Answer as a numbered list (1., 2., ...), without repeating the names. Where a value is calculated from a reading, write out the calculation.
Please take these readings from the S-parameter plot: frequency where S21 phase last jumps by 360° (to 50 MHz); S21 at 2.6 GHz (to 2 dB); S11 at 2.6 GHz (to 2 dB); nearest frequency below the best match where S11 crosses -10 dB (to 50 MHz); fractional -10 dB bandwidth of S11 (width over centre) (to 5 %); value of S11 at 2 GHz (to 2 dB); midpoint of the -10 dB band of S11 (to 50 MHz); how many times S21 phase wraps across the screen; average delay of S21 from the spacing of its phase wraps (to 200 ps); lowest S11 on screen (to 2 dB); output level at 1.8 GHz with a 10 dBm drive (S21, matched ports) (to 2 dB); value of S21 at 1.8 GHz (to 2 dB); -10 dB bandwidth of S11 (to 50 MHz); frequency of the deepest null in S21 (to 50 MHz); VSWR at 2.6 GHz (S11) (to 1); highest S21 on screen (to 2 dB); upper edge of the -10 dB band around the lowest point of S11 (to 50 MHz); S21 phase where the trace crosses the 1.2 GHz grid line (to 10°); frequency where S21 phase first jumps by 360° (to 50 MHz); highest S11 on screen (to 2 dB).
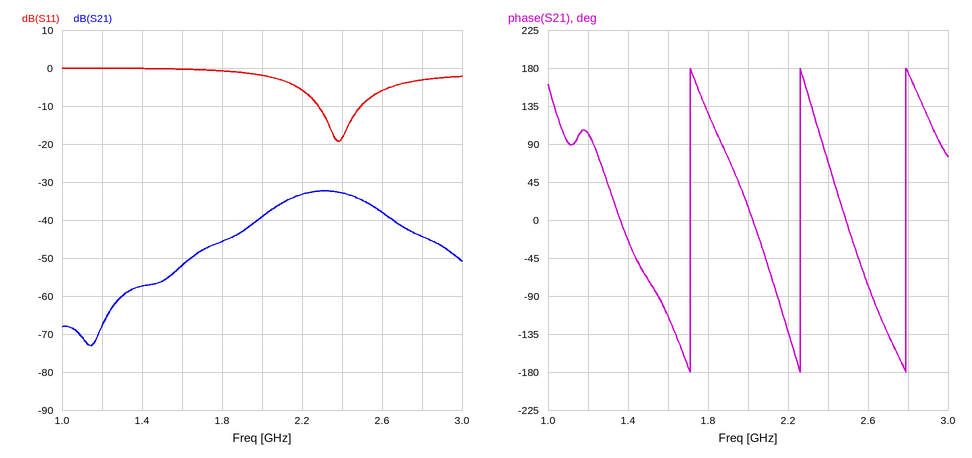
1. 2.80 GHz
2. -38 dB
3. -6 dB
4. 2.30 GHz
5. 200 MHz / 2.4 GHz ≈ 8.33 %, so 10 % to the nearest 5 %
6. -2 dB
7. 2.40 GHz
8. 3
9. 2 cycles / (2.80 GHz − 1.70 GHz) ≈ 1.8 ns
10. -20 dB
11. 10 dBm + (-46 dB) = -36 dBm
12. -46 dB
13. 2.50 GHz − 2.30 GHz = 200 MHz
14. 1.15 GHz
15. |Γ| = 10^(-6/20) = 0.5012; VSWR = (1 + 0.5012)/(1 − 0.5012) ≈ 3
16. -32 dB
17. 2.50 GHz
18. 100°
19. 1.70 GHz
20. 0 dB
